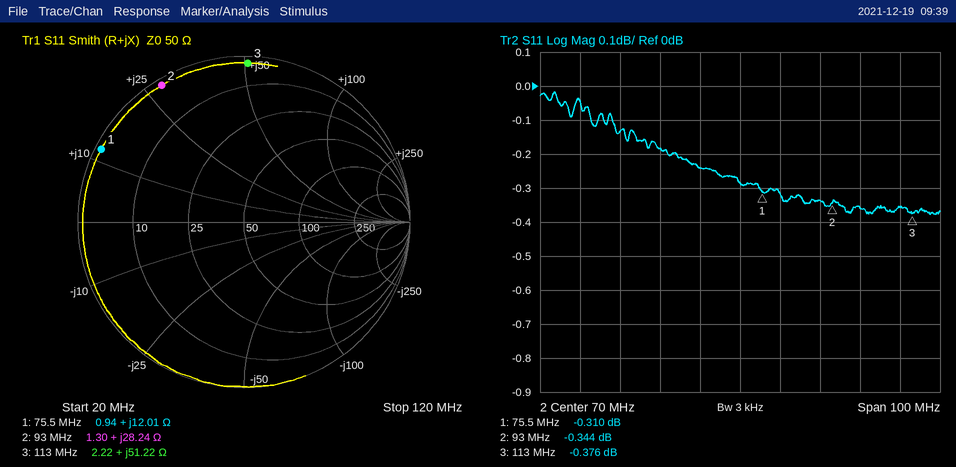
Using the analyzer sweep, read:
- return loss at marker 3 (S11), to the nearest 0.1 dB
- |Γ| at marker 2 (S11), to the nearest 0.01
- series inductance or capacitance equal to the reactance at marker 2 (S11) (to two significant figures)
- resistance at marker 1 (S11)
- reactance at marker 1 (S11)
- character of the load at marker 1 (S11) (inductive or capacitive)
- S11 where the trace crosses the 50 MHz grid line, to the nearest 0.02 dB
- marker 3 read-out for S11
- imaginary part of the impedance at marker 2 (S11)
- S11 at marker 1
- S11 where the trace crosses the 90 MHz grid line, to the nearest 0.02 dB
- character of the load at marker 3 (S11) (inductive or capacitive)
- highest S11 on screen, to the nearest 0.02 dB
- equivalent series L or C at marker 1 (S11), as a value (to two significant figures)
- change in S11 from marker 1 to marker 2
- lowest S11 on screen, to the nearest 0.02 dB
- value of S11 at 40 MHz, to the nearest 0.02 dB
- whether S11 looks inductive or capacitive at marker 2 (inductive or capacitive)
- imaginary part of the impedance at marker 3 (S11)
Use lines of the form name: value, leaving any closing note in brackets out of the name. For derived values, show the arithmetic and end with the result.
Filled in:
return loss at marker 3 (S11), to the nearest 0.1 dB: 0.4 dB
|Γ| at marker 2 (S11), to the nearest 0.01: 0.96
series inductance or capacitance equal to the reactance at marker 2 (S11): L = 28.24 Ω/(2π × 93 MHz) ≈ 48 nH
resistance at marker 1: 0.94 Ω
reactance at marker 1: +12.01 Ω
character of the load at marker 1 (S11): inductive
S11 where the trace crosses the 50 MHz grid line, to the nearest 0.02 dB: -0.18 dB
marker 3 read-out for S11: -0.376 dB
imaginary part of the impedance at marker 2: +28.24 Ω
S11 at marker 1: -0.310 dB
S11 where the trace crosses the 90 MHz grid line, to the nearest 0.02 dB: -0.34 dB
character of the load at marker 3 (S11): inductive
highest S11 on screen, to the nearest 0.02 dB: -0.02 dB
equivalent series L or C at marker 1 (S11), as a value: L = 12.01 Ω/(2π × 75.5 MHz) ≈ 25 nH
change in S11 from marker 1 to marker 2: -0.344 − (-0.31) = -0.034 dB
lowest S11 on screen, to the nearest 0.02 dB: -0.38 dB
value of S11 at 40 MHz, to the nearest 0.02 dB: -0.14 dB
whether S11 looks inductive or capacitive at marker 2: inductive
imaginary part of the impedance at marker 3: +51.22 Ω
